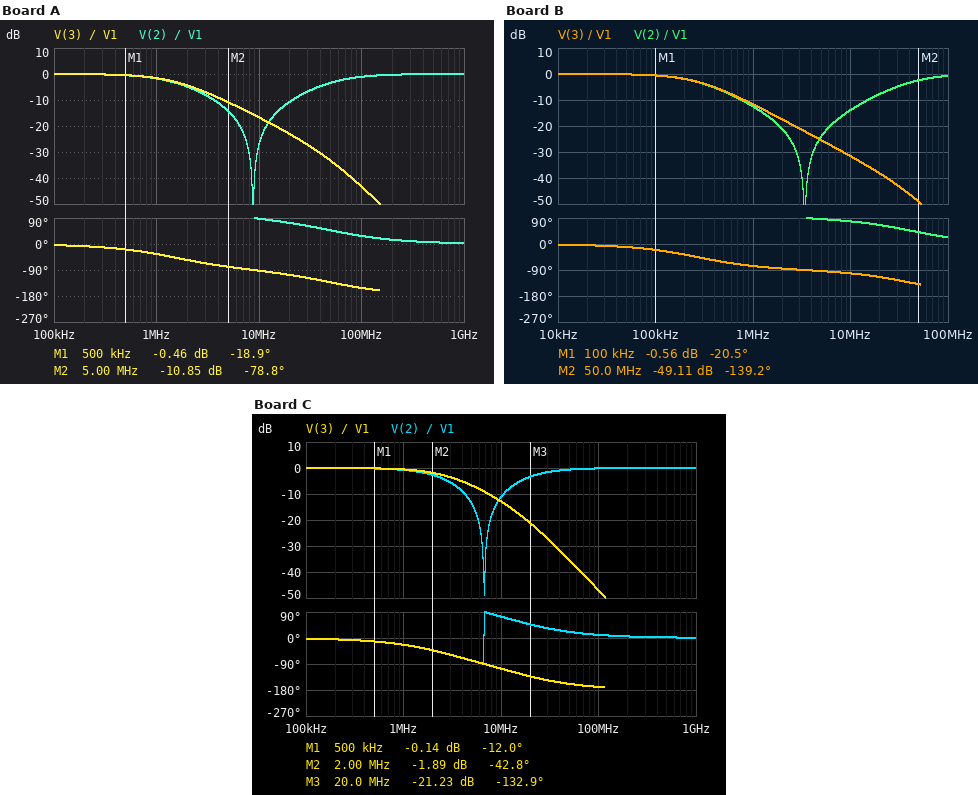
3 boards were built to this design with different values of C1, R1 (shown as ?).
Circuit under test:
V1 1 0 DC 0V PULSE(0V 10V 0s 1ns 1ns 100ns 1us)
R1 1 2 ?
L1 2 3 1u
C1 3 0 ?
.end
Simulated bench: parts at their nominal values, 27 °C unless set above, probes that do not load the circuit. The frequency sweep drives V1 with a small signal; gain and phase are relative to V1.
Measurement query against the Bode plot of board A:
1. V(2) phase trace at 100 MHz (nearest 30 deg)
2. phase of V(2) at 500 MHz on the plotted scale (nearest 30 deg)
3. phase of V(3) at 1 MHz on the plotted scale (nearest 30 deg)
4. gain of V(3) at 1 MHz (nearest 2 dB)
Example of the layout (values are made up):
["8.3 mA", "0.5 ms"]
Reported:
["30 deg", "0 deg", "-30 deg", "-2 dB"]
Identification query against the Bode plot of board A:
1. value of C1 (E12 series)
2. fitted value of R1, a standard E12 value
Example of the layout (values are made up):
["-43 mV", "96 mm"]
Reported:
["330 pF", "330 Ω"]
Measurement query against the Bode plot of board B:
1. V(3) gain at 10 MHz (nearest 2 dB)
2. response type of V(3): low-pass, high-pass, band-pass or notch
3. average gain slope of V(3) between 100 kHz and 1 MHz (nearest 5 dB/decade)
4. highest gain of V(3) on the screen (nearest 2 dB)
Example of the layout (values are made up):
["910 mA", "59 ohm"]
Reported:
["-32 dB", "low-pass", "-10 dB/decade", "0 dB"]
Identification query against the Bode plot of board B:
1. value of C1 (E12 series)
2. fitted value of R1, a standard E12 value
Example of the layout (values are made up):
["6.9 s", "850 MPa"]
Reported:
["2.2 nF", "270 Ω"]
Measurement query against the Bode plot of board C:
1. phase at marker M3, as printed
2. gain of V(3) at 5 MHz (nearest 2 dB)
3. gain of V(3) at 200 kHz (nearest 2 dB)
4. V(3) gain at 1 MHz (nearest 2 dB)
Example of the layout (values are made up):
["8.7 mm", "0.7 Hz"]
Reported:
["-132.9 deg", "-6 dB", "0 dB", "0 dB"]
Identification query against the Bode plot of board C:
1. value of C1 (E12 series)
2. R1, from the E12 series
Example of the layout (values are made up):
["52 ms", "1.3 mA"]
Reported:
["560 pF", "120 Ω"]
